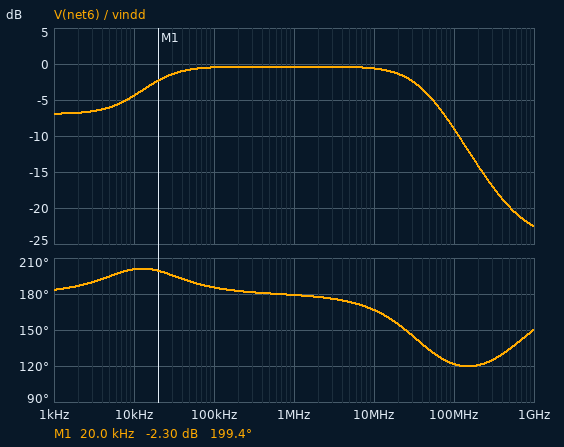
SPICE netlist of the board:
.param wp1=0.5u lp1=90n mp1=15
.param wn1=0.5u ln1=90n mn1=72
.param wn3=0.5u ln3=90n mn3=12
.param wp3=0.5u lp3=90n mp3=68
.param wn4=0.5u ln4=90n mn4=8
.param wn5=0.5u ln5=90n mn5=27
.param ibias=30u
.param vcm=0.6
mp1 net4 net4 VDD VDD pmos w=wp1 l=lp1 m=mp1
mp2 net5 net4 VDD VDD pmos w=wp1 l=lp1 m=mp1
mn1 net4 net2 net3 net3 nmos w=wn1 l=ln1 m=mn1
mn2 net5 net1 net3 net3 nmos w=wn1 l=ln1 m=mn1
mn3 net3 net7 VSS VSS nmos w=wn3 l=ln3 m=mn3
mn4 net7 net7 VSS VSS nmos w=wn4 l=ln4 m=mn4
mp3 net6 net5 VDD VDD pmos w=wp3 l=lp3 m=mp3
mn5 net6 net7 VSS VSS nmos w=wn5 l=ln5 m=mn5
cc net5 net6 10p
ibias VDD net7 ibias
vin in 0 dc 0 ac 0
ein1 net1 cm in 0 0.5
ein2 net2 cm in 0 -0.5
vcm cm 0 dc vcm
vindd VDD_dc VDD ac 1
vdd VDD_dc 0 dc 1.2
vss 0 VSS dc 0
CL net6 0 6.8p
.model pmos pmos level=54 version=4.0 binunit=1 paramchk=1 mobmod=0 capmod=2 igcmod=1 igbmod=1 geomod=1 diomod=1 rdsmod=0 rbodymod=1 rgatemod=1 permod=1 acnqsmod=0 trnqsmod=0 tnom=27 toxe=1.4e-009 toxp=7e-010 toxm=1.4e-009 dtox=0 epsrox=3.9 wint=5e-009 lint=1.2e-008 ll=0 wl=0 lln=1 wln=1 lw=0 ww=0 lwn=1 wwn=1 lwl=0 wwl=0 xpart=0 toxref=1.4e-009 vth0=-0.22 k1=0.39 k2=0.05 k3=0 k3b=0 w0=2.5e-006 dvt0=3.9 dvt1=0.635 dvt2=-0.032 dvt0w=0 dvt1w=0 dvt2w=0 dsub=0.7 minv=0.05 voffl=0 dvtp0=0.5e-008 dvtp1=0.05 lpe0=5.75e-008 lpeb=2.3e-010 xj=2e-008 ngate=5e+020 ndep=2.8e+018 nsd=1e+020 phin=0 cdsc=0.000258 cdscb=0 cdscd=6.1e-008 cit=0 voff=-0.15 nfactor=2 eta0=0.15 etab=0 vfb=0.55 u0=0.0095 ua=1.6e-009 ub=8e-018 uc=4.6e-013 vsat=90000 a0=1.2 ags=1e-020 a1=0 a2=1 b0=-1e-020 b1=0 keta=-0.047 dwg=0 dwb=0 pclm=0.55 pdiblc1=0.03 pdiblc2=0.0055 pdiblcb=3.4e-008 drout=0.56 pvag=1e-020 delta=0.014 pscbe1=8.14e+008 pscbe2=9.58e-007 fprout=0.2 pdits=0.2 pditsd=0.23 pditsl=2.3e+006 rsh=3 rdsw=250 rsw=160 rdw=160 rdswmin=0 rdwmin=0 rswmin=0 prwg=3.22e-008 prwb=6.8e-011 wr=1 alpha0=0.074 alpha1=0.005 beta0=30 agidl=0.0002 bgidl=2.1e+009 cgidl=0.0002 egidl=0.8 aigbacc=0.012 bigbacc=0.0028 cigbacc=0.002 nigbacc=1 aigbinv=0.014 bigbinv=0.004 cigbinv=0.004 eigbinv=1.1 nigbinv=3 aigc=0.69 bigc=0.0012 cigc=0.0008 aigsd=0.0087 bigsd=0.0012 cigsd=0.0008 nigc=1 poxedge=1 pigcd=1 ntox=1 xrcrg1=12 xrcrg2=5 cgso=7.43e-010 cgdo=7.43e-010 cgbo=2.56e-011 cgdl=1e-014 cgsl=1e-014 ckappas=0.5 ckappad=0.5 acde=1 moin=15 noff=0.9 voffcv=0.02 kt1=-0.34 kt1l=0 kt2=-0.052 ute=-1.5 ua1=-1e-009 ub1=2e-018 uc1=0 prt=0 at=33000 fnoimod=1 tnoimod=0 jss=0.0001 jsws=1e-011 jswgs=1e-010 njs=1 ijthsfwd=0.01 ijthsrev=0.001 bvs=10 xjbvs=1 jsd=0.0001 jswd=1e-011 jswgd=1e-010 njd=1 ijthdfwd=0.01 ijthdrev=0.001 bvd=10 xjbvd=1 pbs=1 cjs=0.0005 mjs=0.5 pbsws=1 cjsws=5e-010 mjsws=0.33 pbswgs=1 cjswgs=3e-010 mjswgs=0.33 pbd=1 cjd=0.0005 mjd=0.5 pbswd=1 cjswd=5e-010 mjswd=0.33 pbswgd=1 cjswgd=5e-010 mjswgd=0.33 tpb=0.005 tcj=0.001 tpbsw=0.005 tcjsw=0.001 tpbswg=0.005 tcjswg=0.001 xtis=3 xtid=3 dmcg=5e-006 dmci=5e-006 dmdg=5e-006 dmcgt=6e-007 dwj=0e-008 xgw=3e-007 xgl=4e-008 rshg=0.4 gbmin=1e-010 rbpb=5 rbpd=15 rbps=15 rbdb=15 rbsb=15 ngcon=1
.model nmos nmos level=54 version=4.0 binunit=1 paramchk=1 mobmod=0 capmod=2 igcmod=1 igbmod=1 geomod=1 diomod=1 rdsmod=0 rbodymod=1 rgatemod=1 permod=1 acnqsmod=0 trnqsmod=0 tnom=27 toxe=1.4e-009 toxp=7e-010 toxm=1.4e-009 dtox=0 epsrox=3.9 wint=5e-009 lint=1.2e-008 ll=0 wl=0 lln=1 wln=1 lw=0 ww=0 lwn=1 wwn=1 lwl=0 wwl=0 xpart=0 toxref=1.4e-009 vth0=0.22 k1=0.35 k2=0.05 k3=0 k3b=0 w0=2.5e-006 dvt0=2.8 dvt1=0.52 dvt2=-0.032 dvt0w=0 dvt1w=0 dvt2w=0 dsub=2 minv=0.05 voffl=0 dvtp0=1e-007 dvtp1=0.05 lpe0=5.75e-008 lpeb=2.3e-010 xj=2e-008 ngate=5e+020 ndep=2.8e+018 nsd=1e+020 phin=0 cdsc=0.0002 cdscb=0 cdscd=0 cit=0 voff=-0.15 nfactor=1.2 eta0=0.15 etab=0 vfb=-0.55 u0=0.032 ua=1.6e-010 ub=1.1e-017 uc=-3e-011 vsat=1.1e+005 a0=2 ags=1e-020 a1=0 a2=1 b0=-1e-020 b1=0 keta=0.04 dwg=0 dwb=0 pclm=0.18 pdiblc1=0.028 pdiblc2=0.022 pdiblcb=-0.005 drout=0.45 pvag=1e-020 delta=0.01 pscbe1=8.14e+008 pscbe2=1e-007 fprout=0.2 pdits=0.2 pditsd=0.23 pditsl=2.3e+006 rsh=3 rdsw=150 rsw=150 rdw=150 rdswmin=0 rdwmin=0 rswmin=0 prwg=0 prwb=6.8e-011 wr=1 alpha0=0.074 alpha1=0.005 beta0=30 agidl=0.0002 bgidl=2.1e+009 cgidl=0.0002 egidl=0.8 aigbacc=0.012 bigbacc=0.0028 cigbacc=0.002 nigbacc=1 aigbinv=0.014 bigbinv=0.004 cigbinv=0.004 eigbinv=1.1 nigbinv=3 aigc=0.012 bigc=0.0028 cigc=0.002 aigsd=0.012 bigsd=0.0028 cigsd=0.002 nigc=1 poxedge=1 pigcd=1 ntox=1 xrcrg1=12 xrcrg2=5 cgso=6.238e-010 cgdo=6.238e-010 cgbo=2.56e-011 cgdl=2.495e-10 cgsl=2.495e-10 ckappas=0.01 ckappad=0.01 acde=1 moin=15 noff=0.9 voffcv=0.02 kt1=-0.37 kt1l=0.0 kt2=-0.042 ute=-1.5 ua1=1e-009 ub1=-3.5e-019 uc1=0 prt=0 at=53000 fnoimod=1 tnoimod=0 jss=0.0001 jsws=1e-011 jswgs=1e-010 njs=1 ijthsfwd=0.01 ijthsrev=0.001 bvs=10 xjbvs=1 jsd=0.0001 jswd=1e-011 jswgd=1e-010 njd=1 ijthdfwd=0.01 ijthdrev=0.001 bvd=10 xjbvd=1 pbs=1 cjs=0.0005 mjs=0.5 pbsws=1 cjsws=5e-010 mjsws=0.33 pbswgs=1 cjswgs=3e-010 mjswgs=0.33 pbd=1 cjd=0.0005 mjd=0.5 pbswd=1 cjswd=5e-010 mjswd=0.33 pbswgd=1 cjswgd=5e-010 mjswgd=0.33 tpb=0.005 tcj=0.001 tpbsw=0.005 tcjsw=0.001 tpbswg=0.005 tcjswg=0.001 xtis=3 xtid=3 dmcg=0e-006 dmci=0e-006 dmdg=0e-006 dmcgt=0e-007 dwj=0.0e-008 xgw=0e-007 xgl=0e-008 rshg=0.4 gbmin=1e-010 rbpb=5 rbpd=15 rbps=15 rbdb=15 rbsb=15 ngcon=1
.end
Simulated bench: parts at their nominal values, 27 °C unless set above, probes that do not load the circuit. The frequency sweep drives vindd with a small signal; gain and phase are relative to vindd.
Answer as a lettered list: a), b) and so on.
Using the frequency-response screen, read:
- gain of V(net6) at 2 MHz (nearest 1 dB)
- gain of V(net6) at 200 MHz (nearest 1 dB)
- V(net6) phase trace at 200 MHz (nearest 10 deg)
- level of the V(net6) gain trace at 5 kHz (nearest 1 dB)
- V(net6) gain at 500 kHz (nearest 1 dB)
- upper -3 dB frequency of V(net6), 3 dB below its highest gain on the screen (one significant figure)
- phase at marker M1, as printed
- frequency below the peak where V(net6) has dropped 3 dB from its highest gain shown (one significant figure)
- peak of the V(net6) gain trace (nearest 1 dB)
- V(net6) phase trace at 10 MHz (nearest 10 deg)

a) 0 dB
b) -14 dB
c) 120 deg
d) -6 dB
e) 0 dB
f) 40 MHz
g) 199.4 deg
h) 10 kHz
i) 0 dB
j) 170 deg
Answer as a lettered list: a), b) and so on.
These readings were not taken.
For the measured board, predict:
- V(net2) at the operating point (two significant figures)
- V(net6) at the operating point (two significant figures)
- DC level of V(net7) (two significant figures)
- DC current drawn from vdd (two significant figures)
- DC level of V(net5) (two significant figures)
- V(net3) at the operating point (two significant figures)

a) 600 mV
b) 520 mV
c) 390 mV
d) 180 µA
e) 820 mV
f) 340 mV
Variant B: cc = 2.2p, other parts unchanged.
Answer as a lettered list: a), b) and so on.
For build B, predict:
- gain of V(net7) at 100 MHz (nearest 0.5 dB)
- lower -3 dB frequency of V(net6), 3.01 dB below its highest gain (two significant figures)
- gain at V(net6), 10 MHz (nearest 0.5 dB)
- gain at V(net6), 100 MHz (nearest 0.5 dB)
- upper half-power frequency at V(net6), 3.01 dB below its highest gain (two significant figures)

a) -46.5 dB
b) 59 kHz
c) -1.0 dB
d) -9.5 dB
e) 38 MHz
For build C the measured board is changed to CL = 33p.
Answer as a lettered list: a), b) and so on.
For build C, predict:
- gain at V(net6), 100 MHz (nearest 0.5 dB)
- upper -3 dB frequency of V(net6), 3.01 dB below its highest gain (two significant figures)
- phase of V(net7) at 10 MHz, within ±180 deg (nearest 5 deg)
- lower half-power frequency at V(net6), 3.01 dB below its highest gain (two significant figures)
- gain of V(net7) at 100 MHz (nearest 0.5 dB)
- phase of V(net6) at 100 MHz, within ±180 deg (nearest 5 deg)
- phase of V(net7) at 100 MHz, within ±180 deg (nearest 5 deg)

a) -21.5 dB
b) 8.8 MHz
c) -145 deg
d) 13 kHz
e) -58.5 dB
f) 105 deg
g) -165 deg
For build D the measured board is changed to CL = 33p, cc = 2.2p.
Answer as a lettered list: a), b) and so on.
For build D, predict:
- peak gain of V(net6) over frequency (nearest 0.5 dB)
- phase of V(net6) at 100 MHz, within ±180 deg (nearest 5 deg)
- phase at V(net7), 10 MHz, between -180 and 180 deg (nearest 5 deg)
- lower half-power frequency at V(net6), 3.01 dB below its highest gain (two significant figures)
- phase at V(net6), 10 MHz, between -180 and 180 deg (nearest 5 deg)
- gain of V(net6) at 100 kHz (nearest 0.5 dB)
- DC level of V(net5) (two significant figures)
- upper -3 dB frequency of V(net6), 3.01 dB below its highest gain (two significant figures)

a) -2.0 dB
b) 105 deg
c) -140 deg
d) 44 kHz
e) 135 deg
f) -3.0 dB
g) 820 mV
h) 9.5 MHz
